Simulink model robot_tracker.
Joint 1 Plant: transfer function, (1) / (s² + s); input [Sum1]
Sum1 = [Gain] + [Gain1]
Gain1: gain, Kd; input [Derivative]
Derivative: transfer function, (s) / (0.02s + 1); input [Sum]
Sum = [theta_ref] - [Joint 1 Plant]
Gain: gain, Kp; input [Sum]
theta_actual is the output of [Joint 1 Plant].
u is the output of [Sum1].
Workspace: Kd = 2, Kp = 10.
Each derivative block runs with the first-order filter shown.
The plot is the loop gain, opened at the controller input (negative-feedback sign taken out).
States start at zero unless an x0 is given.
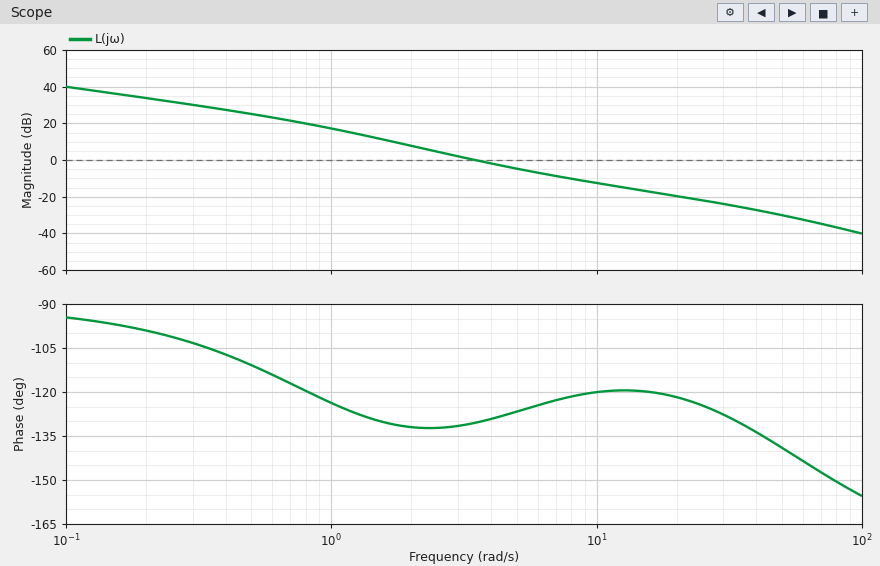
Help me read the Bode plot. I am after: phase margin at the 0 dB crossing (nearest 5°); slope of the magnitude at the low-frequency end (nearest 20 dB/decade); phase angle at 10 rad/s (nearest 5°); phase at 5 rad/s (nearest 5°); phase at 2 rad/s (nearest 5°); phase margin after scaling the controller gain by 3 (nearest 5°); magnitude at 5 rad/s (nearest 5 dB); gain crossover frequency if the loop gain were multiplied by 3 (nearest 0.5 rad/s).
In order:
50°
-20 dB/decade
-120°
-125°
-130°
60°
-5 dB
7.5 rad/s
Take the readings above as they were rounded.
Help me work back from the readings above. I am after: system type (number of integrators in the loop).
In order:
1
